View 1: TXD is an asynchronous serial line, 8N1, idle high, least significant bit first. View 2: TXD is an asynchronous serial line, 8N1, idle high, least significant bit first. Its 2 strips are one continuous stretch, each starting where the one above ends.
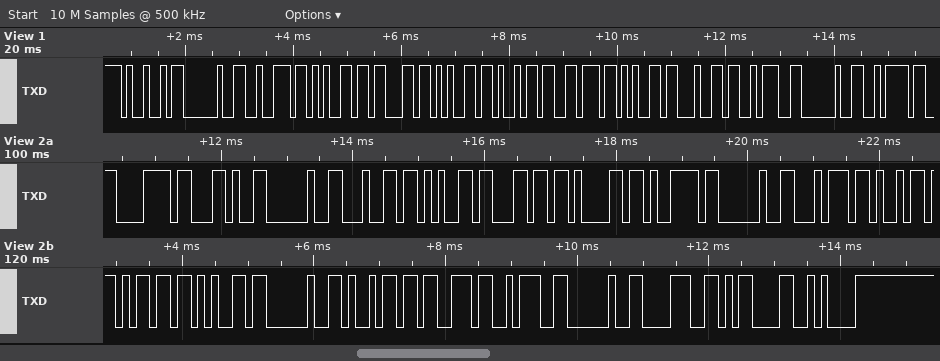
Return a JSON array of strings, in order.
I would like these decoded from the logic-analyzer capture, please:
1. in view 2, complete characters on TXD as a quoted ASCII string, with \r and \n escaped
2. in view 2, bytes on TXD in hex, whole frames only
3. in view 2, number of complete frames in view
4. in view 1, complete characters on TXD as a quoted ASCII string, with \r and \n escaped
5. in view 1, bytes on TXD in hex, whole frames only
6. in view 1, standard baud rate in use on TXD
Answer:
["\"x, delay time is: 8\\r\\n\"", "78 2C 20 64 65 6C 61 79 20 74 69 6D 65 20 69 73 3A 20 38 0D 0A", "21", "\"I received: z\"", "49 20 72 65 63 65 69 76 65 64 3A 20 7A", "9600 baud"]
